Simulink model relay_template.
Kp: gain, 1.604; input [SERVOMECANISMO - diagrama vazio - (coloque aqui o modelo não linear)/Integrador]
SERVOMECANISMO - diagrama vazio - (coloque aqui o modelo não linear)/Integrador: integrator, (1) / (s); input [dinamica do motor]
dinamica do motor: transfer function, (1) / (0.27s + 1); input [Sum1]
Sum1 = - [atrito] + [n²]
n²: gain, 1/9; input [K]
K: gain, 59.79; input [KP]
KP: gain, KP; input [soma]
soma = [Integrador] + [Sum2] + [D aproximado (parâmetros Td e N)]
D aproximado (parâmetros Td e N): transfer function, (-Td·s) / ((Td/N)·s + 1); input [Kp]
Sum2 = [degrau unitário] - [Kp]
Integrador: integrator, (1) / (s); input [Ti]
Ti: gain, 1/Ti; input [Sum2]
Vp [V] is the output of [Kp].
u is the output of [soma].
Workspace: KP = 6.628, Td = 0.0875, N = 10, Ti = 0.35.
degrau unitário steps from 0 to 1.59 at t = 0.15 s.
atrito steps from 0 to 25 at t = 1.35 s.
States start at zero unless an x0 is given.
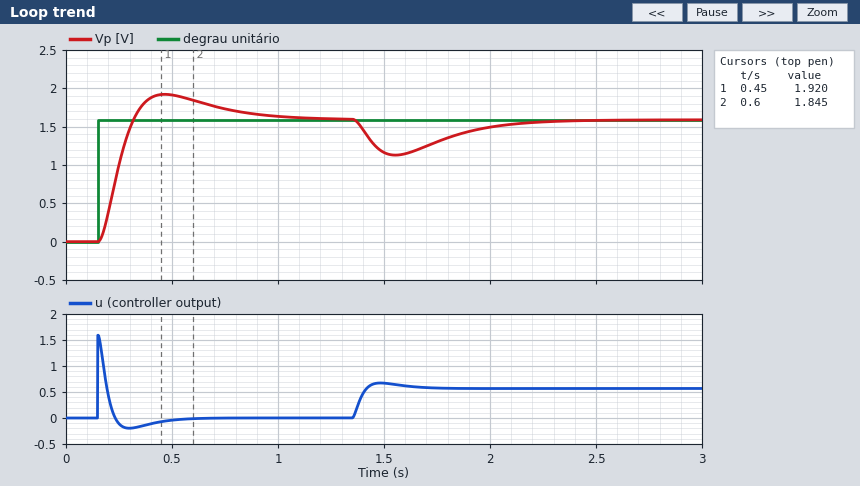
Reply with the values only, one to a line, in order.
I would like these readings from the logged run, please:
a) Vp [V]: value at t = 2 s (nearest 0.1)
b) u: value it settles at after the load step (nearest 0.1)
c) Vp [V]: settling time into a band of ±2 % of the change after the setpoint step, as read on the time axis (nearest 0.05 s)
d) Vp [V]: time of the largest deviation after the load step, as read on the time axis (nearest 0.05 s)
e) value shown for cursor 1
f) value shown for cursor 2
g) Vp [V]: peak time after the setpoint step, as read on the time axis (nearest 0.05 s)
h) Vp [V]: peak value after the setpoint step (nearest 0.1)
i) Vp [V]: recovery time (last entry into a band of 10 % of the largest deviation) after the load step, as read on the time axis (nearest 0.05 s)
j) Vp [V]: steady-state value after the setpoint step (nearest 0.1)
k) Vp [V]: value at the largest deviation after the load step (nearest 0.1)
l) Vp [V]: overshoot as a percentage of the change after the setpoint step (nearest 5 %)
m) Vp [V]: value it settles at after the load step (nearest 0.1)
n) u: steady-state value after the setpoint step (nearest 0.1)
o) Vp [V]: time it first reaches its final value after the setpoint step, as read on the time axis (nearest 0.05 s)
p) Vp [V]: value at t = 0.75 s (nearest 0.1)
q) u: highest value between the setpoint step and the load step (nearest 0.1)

1.5
0.6
1.05 s
1.55 s
1.920
1.845
0.45 s
1.9
2.15 s
1.6
1.1
20 %
1.6
0.0
0.30 s
1.7
1.6
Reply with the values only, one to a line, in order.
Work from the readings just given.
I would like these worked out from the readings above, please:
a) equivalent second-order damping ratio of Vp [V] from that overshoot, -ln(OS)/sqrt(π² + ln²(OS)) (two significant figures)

0.46
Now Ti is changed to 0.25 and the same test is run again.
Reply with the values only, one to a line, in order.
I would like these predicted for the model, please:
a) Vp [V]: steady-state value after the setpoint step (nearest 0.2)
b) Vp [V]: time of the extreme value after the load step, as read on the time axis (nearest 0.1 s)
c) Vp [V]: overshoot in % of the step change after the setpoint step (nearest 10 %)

1.6
1.5 s
30 %
